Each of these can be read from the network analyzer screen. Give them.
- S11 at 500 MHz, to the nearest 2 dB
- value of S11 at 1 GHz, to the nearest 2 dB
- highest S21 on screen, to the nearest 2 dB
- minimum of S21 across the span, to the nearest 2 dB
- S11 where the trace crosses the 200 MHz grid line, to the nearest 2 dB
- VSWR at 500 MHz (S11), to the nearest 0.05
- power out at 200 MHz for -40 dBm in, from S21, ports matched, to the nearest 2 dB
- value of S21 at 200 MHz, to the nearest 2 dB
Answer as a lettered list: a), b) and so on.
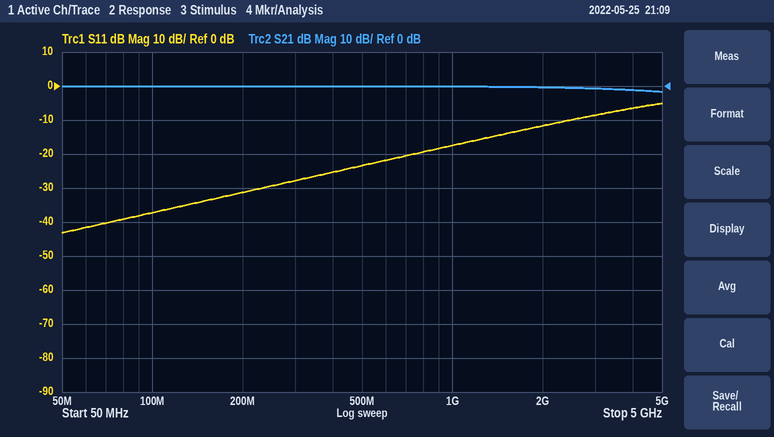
a) -24 dB
b) -18 dB
c) 0 dB
d) -2 dB
e) -32 dB
f) 1.15
g) -40 dBm
h) 0 dB
